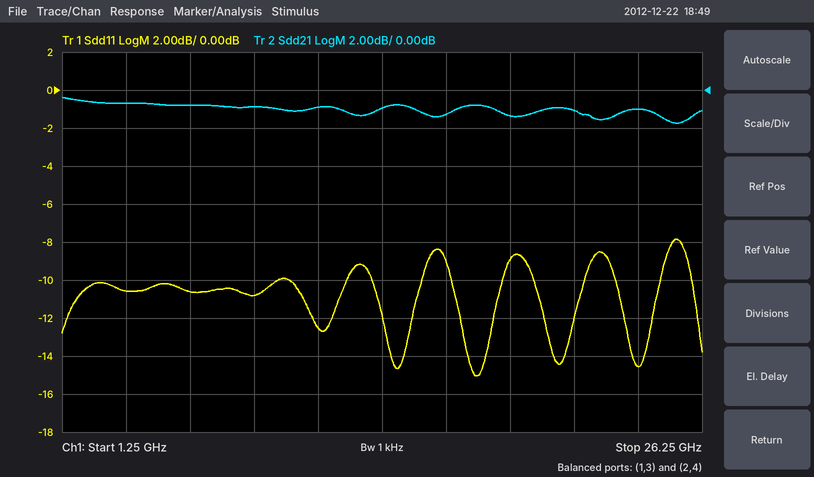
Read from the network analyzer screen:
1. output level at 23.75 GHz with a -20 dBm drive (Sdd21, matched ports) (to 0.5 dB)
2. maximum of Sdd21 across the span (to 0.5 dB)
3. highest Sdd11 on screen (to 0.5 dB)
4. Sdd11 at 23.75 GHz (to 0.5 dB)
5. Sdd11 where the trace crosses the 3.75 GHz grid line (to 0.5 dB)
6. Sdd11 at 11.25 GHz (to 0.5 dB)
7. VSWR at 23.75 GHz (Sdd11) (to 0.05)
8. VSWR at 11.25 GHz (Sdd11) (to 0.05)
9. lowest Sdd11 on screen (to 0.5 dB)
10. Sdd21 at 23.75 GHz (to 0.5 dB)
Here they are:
-21.0 dBm
-0.5 dB
-8.0 dB
-14.5 dB
-10.5 dB
-12.5 dB
1.45
1.60
-15.0 dB
-1.0 dB
